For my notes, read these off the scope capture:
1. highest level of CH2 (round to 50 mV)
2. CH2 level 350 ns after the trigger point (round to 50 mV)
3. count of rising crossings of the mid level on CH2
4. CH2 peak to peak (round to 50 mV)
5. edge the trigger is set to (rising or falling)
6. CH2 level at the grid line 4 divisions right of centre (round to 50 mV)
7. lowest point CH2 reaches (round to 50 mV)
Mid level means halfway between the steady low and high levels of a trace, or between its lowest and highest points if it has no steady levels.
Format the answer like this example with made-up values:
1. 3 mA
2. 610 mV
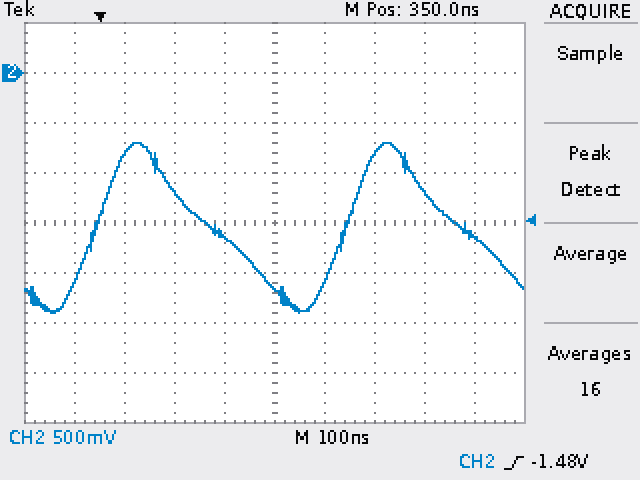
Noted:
1. -700 mV
2. -2.15 V
3. 2
4. 1.70 V
5. rising
6. -1.65 V
7. -2.40 V
